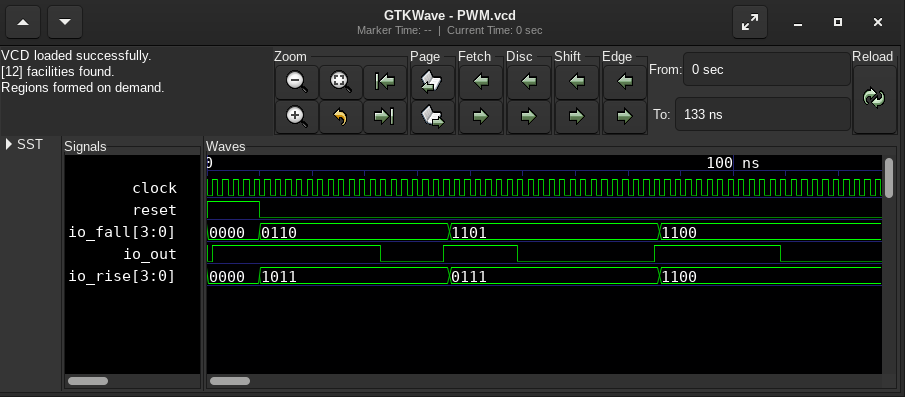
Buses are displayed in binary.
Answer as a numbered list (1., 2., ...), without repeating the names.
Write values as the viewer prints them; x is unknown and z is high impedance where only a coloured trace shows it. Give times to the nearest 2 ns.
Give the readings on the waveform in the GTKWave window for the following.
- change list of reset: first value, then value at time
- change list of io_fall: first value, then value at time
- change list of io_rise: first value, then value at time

1. 1, 0 at 10 ns
2. 0000, 0110 at 10 ns, 1101 at 46 ns, 1100 at 86 ns
3. 0000, 1011 at 10 ns, 0111 at 46 ns, 1100 at 86 ns
